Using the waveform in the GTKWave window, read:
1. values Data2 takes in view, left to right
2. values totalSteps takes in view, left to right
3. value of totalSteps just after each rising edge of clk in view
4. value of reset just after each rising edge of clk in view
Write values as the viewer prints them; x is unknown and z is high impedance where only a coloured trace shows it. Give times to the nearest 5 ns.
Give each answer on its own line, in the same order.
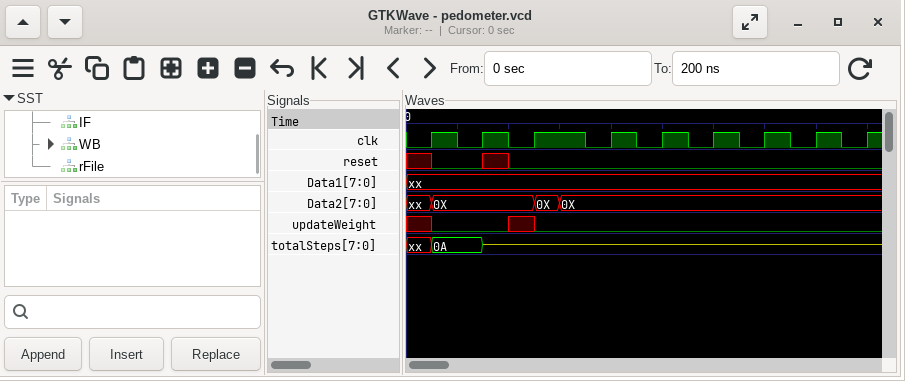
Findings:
xx, 0X, 0X, 0X
xx, 0A, z
0A, z, z, z, z, z, z, z, z
0 x 0 0 0 0 0 0 0
